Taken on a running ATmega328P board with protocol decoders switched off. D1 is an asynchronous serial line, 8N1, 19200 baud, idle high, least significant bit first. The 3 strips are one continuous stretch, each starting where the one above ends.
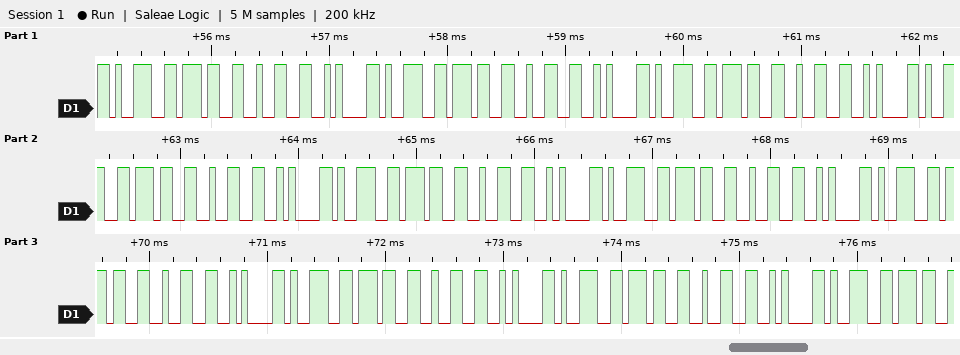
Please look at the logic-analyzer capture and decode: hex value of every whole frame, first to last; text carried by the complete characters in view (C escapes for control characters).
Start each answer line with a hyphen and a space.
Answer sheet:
- 39 37 32 0A 39 37 32 0A 39 37 32 0A 39 37 32 0A 39 37 32 0A 39 37 32 0A 39 37 32 0A 39 37 32 0A 39 37 32 0A 39 37
- "972\n972\n972\n972\n972\n972\n972\n972\n972\n97"
